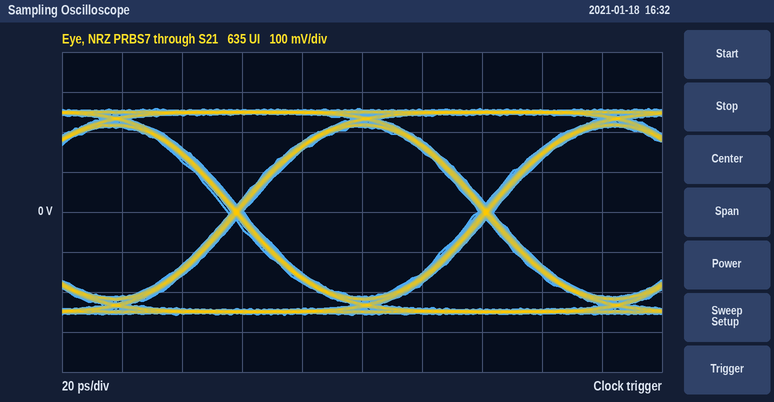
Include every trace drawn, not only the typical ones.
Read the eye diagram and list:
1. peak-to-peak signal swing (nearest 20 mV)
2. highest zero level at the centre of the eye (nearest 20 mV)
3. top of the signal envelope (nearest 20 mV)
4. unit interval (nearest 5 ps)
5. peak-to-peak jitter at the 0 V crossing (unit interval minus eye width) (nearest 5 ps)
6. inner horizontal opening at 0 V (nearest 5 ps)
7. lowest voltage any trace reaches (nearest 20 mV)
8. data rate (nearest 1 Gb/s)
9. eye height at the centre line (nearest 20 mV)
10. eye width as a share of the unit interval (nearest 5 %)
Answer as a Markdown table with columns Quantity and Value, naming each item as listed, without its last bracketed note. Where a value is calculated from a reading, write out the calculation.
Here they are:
| Quantity | Value |
|---|---|
| peak-to-peak signal swing | 520 mV |
| highest zero level at the centre of the eye | -220 mV |
| top of the signal envelope | 260 mV |
| unit interval | 85 ps |
| peak-to-peak jitter at the 0 V crossing (unit interval minus eye width) | 5 ps |
| inner horizontal opening at 0 V | 80 ps |
| lowest voltage any trace reaches | -260 mV |
| data rate | 12 Gb/s |
| eye height at the centre line | 420 mV |
| eye width as a share of the unit interval | 80 ps / 85 ps ≈ 94.1 %, so 95 % to the nearest 5 % |
